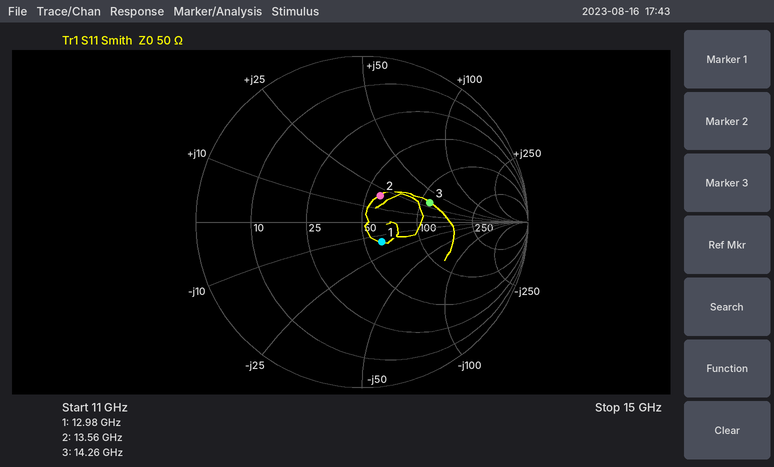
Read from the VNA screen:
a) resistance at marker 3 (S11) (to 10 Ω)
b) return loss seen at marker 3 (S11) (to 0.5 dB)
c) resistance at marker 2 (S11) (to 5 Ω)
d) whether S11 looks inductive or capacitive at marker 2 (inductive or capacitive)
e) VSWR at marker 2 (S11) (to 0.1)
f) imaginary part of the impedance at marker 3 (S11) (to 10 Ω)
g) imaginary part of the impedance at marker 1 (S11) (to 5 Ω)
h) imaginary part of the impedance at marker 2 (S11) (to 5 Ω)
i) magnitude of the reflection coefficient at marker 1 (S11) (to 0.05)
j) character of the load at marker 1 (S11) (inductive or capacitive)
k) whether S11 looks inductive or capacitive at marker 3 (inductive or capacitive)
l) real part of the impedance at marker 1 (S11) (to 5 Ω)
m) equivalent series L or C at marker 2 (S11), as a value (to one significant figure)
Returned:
110 Ω
7.5 dB
60 Ω
inductive
1.5
+30 Ω
-15 Ω
+20 Ω
0.15
capacitive
inductive
60 Ω
200 pH
